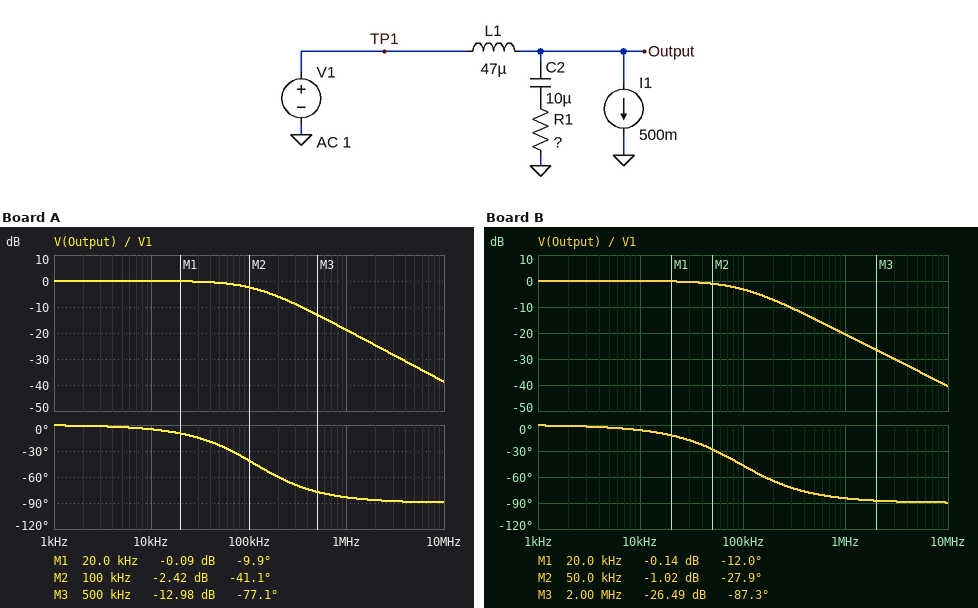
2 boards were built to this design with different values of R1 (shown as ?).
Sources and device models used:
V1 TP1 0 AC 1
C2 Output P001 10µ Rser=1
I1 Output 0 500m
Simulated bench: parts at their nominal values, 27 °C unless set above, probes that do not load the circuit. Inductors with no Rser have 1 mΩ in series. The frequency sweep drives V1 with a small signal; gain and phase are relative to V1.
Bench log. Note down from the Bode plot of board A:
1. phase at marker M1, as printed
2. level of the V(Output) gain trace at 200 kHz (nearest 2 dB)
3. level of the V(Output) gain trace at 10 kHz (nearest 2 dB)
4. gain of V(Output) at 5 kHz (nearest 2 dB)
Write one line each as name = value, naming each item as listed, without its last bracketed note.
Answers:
phase at marker M1, as printed = -9.9 deg
level of the V(Output) gain trace at 200 kHz = -6 dB
level of the V(Output) gain trace at 10 kHz = 0 dB
gain of V(Output) at 5 kHz = 0 dB
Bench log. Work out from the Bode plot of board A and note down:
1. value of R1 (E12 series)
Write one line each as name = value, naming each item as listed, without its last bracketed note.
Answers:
value of R1 = 33 Ω
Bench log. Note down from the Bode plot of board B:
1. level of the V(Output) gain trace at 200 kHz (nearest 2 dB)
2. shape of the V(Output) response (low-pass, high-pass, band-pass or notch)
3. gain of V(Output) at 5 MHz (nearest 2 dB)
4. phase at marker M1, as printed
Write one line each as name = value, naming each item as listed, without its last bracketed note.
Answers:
level of the V(Output) gain trace at 200 kHz = -8 dB
shape of the V(Output) response = low-pass
gain of V(Output) at 5 MHz = -34 dB
phase at marker M1, as printed = -12.0 deg
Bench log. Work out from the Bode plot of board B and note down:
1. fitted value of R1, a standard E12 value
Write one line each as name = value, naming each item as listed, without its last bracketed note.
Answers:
fitted value of R1, a standard E12 value = 27 Ω
